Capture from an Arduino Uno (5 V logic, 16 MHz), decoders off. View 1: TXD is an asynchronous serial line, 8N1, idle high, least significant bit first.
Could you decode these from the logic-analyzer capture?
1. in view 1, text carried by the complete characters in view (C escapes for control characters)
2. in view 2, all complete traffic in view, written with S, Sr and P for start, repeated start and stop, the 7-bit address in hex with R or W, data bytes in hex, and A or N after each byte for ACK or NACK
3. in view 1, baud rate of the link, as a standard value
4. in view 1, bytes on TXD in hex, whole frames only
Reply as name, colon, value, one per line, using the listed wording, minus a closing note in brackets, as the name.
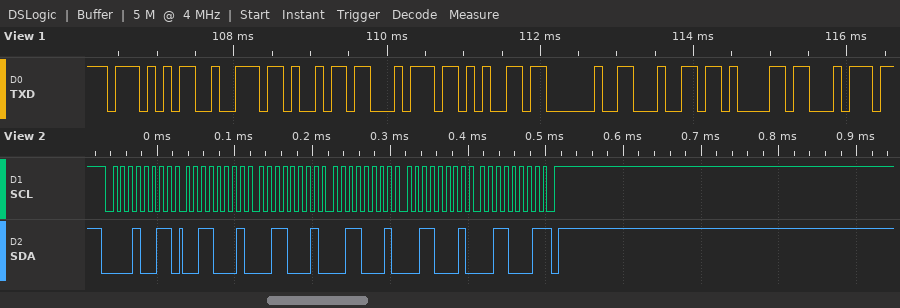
in view 1, text carried by the complete characters in view: "Write dat"
in view 2, all complete traffic in view, written with S, Sr and P for start, repeated start and stop, the 7-bit address in hex with R or W, data bytes in hex, and A or N after each byte for ACK or NACK: S 09R A 31 A 31 A 31 A 31 A 31 N P
in view 1, baud rate of the link, as a standard value: 9600 baud
in view 1, bytes on TXD in hex, whole frames only: 57 72 69 74 65 20 64 61 74
